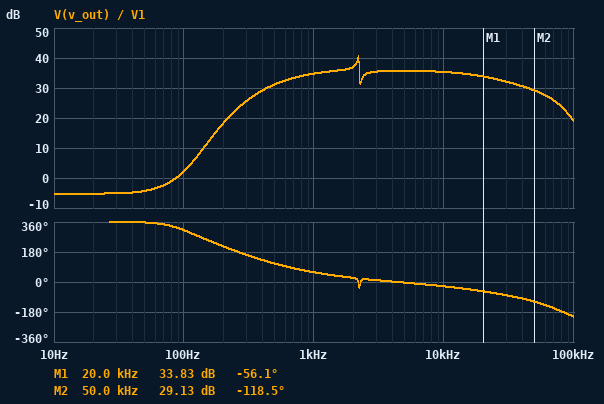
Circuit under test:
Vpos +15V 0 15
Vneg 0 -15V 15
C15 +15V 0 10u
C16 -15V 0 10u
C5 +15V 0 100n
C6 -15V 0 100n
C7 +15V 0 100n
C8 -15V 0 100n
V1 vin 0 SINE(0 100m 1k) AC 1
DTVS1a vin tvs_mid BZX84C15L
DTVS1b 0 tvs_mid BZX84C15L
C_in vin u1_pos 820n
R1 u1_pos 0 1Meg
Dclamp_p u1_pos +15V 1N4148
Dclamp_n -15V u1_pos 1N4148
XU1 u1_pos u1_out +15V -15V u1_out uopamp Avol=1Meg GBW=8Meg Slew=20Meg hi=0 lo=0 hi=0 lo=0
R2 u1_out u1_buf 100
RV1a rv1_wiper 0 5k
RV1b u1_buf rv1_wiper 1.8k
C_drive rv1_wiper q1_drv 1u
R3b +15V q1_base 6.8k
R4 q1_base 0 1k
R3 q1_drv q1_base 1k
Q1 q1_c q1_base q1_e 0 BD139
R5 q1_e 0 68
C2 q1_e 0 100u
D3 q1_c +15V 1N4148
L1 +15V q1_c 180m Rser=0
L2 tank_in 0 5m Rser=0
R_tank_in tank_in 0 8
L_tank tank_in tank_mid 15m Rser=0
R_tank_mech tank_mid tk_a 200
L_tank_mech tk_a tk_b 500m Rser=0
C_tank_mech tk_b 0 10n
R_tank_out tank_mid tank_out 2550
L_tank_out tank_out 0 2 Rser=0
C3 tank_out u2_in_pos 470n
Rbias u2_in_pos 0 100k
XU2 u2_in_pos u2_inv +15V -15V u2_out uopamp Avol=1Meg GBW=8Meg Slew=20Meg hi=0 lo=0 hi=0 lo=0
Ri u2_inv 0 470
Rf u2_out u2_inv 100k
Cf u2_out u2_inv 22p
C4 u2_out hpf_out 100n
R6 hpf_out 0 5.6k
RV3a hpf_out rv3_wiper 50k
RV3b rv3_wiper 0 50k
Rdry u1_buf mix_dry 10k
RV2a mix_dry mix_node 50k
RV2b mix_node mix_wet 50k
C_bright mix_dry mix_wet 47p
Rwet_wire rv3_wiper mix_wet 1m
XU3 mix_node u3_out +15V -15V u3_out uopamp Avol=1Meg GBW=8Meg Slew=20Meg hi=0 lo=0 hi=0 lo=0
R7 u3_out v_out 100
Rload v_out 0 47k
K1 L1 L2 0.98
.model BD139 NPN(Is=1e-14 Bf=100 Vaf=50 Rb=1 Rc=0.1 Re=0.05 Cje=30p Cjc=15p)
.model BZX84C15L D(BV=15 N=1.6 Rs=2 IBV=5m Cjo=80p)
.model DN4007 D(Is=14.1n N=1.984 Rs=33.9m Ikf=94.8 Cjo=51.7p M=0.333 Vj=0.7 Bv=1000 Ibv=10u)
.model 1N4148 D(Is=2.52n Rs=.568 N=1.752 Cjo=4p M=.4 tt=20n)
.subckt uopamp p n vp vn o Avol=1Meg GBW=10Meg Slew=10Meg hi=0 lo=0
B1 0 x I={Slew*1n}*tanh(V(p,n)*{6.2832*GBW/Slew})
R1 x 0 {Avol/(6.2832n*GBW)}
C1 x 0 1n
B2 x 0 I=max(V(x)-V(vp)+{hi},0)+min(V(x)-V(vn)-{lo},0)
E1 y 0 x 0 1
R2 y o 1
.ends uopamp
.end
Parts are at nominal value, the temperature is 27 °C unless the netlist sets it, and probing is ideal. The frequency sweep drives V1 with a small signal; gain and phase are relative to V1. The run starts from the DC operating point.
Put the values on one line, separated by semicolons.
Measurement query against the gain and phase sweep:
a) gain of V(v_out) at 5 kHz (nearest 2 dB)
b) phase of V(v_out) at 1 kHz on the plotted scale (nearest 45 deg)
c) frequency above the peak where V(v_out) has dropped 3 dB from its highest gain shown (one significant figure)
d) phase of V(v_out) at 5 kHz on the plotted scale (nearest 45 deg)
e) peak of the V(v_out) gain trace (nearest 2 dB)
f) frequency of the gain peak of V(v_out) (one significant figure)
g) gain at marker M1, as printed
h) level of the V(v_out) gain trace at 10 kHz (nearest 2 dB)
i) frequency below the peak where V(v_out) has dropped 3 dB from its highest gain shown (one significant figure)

36 dB; 45 deg; 2 kHz; 0 deg; 40 dB; 2 kHz; 33.83 dB; 36 dB; 2 kHz
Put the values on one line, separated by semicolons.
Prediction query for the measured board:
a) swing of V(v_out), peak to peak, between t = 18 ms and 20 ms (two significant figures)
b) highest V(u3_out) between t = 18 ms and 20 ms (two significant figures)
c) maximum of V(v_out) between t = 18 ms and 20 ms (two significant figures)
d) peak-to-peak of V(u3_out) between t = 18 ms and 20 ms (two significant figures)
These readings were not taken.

8.0 V; 4.1 V; 4.1 V; 8.0 V
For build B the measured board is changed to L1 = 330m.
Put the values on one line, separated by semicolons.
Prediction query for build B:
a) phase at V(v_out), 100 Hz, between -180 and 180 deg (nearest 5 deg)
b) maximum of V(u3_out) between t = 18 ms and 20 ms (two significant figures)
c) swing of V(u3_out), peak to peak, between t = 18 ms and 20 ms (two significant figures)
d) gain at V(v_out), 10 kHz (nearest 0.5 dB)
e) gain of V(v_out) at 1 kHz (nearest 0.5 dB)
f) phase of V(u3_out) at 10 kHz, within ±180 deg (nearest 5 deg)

-55 deg; 4.4 V; 8.1 V; 37.5 dB; 37.0 dB; -30 deg
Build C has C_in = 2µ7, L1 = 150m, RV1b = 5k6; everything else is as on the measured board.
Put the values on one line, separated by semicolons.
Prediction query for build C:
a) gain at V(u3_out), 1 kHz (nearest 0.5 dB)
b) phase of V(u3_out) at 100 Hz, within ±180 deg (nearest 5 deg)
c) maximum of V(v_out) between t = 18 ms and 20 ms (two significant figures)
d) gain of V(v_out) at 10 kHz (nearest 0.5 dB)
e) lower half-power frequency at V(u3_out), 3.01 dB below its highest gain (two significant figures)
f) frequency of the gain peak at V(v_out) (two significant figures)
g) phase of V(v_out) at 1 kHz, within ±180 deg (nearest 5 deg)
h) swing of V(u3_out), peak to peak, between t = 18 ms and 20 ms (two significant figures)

26.5 dB; -35 deg; 2.1 V; 27.0 dB; 2.0 kHz; 2.2 kHz; 55 deg; 4.3 V
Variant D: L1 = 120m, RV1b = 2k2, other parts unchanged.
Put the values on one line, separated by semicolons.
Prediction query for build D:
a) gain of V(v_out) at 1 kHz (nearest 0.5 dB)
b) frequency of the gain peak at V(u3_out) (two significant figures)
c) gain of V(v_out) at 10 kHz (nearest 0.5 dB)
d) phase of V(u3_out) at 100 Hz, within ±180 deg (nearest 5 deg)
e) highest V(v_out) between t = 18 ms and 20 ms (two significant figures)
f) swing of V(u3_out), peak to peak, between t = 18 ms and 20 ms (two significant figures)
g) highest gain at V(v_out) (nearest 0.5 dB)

32.0 dB; 2.2 kHz; 32.5 dB; -45 deg; 3.7 V; 7.3 V; 37.5 dB
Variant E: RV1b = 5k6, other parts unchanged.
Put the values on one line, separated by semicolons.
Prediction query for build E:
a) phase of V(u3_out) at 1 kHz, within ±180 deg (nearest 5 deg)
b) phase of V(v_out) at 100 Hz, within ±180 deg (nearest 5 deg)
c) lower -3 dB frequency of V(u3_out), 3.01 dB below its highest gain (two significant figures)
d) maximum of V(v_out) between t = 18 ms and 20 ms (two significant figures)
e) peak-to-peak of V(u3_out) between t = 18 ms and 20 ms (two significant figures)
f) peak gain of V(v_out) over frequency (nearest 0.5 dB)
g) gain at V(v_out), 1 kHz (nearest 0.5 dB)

55 deg; -40 deg; 2.0 kHz; 2.3 V; 4.7 V; 32.5 dB; 27.5 dB
